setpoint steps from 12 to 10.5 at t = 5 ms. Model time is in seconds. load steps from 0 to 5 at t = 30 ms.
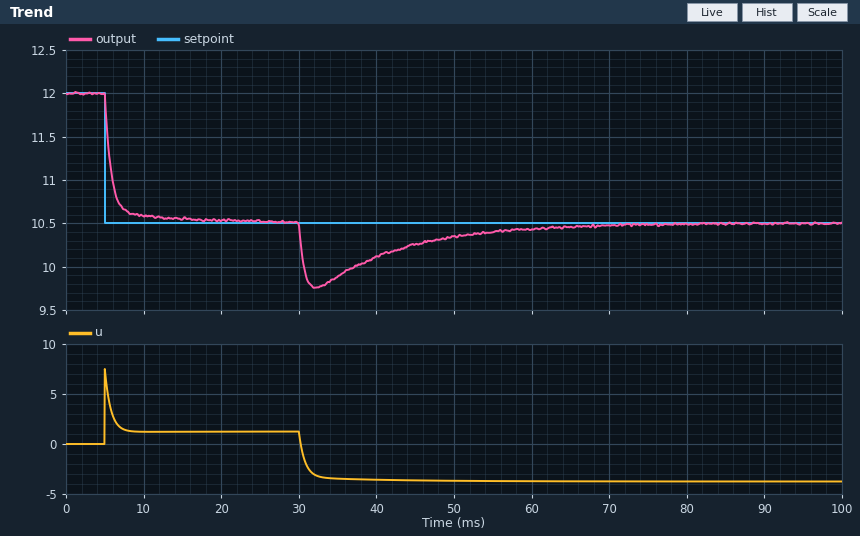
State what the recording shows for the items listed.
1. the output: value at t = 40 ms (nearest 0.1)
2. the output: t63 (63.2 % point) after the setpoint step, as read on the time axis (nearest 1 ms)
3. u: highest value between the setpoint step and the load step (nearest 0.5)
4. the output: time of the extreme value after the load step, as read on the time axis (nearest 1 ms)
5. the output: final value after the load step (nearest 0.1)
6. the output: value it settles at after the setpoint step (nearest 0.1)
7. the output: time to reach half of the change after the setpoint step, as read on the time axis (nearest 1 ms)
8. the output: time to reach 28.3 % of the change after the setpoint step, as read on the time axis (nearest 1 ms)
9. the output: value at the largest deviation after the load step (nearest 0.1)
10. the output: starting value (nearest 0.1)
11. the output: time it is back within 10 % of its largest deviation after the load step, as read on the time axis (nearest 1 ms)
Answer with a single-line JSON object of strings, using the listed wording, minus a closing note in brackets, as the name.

{"the output: value at t = 40 ms": "10.1", "the output: t63 (63.2 % point) after the setpoint step, as read on the time axis": "6 ms", "u: highest value between the setpoint step and the load step": "7.5", "the output: time of the extreme value after the load step, as read on the time axis": "32 ms", "the output: final value after the load step": "10.5", "the output: value it settles at after the setpoint step": "10.5", "the output: time to reach half of the change after the setpoint step, as read on the time axis": "6 ms", "the output: time to reach 28.3 % of the change after the setpoint step, as read on the time axis": "5 ms", "the output: value at the largest deviation after the load step": "9.8", "the output: starting value": "12.0", "the output: time it is back within 10 % of its largest deviation after the load step, as read on the time axis": "58 ms"}
